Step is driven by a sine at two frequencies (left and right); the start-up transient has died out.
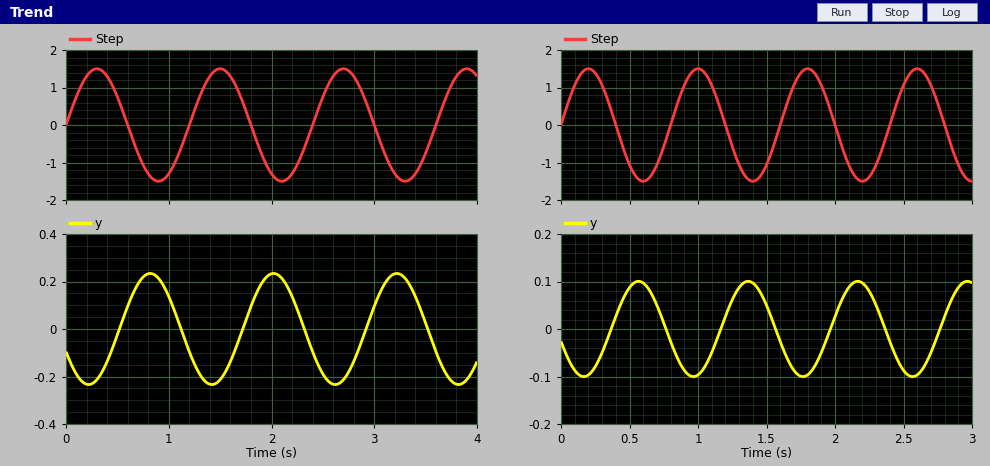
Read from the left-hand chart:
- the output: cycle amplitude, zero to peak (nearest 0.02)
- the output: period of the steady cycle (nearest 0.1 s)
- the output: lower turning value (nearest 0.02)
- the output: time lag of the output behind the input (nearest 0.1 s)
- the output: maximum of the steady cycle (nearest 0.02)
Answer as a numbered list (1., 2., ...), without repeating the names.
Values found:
1. 0.24
2. 1.2 s
3. -0.24
4. 0.5 s
5. 0.24
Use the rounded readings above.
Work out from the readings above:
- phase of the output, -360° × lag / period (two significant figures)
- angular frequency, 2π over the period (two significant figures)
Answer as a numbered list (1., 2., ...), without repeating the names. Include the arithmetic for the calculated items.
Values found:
1. -360 × 0.5 / 1.2 = -150°
2. 2π / 1.2 = 5.2 rad/s
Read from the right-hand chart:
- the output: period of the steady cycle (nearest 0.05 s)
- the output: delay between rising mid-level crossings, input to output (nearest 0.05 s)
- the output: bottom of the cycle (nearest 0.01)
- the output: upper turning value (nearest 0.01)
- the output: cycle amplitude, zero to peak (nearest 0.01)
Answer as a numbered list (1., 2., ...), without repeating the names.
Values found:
1. 0.80 s
2. 0.35 s
3. -0.10
4. 0.10
5. 0.10
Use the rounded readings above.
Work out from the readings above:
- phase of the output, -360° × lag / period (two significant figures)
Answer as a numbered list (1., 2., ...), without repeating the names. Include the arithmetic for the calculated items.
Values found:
1. -360 × 0.35 / 0.8 = -160°
